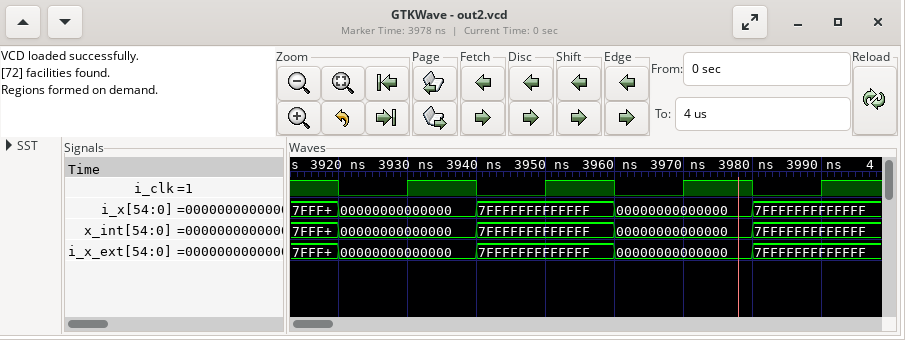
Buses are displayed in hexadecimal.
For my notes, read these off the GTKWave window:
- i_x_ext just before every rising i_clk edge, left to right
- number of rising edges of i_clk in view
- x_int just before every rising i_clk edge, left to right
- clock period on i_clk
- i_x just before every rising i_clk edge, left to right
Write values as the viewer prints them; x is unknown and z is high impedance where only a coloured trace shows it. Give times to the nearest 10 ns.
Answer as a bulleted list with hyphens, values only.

- 00000000000000, 7FFFFFFFFFFFFF, 00000000000000, 7FFFFFFFFFFFFF
- 4
- 00000000000000, 7FFFFFFFFFFFFF, 00000000000000, 7FFFFFFFFFFFFF
- 20 ns
- 00000000000000, 7FFFFFFFFFFFFF, 00000000000000, 7FFFFFFFFFFFFF
